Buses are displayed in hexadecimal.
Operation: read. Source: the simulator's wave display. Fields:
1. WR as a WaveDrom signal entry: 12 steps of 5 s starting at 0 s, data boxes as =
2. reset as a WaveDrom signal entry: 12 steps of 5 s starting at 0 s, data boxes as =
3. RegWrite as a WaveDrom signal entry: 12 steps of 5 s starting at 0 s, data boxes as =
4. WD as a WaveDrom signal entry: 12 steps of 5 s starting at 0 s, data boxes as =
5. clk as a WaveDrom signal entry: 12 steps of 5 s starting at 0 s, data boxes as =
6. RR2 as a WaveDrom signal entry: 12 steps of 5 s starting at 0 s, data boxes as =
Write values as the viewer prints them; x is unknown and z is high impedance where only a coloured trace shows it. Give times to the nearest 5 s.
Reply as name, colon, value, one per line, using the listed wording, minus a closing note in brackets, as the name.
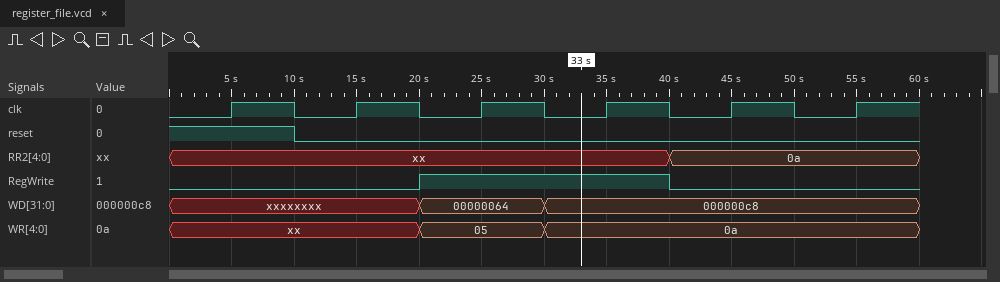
WR as a WaveDrom signal entry: 12 steps of 5 s starting at 0 s, data boxes as =: {name: 'WR', wave: 'x...=.=.....', data: '05 0a'}
reset as a WaveDrom signal entry: 12 steps of 5 s starting at 0 s, data boxes as =: {name: 'reset', wave: '1.0.........'}
RegWrite as a WaveDrom signal entry: 12 steps of 5 s starting at 0 s, data boxes as =: {name: 'RegWrite', wave: '0...1...0...'}
WD as a WaveDrom signal entry: 12 steps of 5 s starting at 0 s, data boxes as =: {name: 'WD', wave: 'x...=.=.....', data: '00000064 000000c8'}
clk as a WaveDrom signal entry: 12 steps of 5 s starting at 0 s, data boxes as =: {name: 'clk', wave: '010101010101'}
RR2 as a WaveDrom signal entry: 12 steps of 5 s starting at 0 s, data boxes as =: {name: 'RR2', wave: 'x.......=...', data: '0a'}
